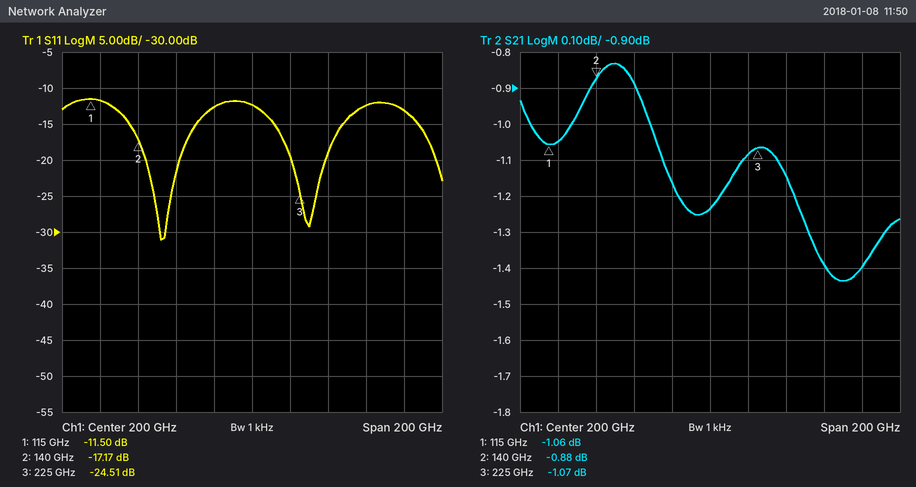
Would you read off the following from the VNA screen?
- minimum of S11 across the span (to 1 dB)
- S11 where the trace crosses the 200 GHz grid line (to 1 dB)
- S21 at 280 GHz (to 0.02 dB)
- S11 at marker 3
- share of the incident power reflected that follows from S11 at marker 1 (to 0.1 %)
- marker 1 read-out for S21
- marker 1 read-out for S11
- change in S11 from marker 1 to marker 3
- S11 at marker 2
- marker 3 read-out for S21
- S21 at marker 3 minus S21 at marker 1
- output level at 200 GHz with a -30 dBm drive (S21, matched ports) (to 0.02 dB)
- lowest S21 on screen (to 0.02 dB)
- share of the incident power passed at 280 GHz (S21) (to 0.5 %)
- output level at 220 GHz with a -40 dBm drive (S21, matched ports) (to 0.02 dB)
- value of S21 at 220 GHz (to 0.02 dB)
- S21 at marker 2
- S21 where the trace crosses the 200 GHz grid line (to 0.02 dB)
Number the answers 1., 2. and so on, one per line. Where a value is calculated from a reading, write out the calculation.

1. -31 dB
2. -12 dB
3. -1.40 dB
4. -24.51 dB
5. 10^(-11.5/10) ≈ 7.1 %
6. -1.06 dB
7. -11.50 dB
8. -24.51 − (-11.5) = -13.01 dB
9. -17.17 dB
10. -1.07 dB
11. -1.07 − (-1.06) = -0.01 dB
12. -30 dBm + (-1.24 dB) = -31.24 dBm
13. -1.44 dB
14. 10^(-1.4/10) ≈ 72.4 %, so 72.5 % to the nearest 0.5 %
15. -40 dBm + (-1.08 dB) = -41.08 dBm
16. -1.08 dB
17. -0.88 dB
18. -1.24 dB
